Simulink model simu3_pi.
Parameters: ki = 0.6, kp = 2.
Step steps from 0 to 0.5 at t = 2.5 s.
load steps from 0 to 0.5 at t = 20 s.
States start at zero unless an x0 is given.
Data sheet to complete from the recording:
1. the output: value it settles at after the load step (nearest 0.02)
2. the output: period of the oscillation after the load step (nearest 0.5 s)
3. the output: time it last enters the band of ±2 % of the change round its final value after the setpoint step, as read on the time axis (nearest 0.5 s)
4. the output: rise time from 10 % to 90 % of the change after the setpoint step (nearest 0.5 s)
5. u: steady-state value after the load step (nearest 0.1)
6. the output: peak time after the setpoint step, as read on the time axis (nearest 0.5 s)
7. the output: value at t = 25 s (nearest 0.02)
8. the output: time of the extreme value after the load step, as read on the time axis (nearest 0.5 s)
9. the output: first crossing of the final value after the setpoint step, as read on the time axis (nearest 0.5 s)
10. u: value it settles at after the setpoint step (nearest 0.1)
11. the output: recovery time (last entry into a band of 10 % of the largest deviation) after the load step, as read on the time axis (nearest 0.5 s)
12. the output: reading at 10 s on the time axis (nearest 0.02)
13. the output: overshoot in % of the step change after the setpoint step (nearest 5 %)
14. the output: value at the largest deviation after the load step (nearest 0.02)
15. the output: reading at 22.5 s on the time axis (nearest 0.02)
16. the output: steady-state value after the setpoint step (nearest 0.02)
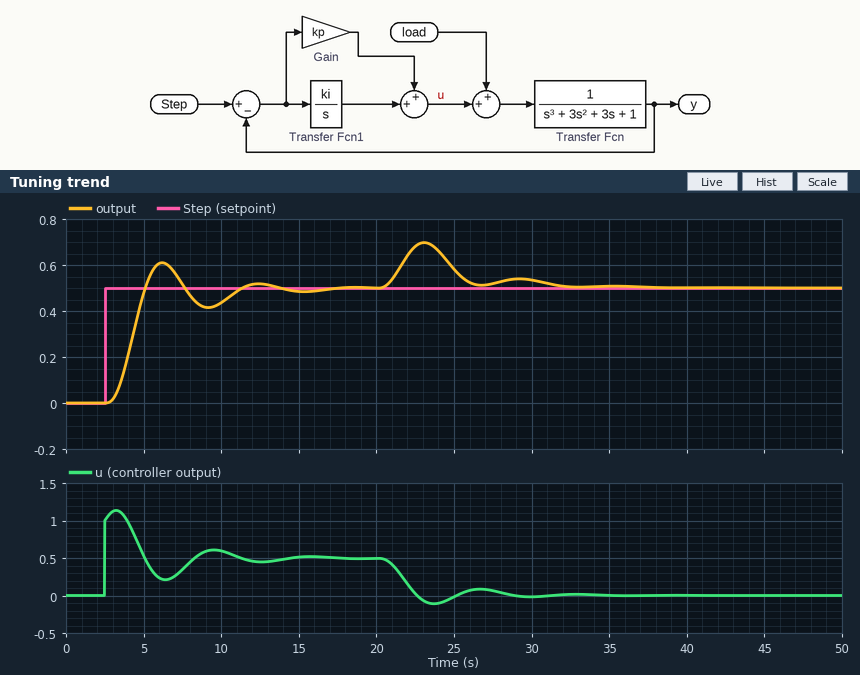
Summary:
0.50
6.0 s
16.5 s
1.5 s
0.0
6.0 s
0.58
23.0 s
5.0 s
0.5
31.0 s
0.44
20 %
0.70
0.68
0.50
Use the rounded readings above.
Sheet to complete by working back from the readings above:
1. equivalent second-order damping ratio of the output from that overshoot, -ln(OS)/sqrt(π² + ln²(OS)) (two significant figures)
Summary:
0.46
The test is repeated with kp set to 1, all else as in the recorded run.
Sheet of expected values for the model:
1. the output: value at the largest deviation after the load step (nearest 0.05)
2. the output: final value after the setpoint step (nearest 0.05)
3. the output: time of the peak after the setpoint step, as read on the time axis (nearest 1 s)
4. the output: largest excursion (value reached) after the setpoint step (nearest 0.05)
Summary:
0.75
0.50
8 s
0.60
